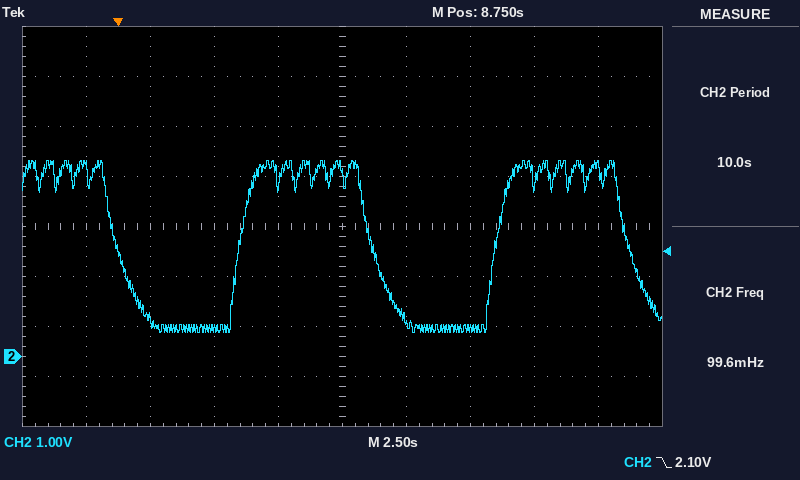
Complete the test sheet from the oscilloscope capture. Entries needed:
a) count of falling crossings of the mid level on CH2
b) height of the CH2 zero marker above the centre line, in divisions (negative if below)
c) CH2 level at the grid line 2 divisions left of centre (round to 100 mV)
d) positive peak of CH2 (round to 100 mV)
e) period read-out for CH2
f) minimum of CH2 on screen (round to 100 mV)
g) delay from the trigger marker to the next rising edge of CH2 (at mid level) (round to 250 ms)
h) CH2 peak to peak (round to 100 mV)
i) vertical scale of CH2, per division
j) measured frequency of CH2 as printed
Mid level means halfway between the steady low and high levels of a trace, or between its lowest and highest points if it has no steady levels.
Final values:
3
-2.6 div
600 mV
3.9 V
10.0 s
500 mV
4.75 s
3.4 V
1 V
99.6 mHz
